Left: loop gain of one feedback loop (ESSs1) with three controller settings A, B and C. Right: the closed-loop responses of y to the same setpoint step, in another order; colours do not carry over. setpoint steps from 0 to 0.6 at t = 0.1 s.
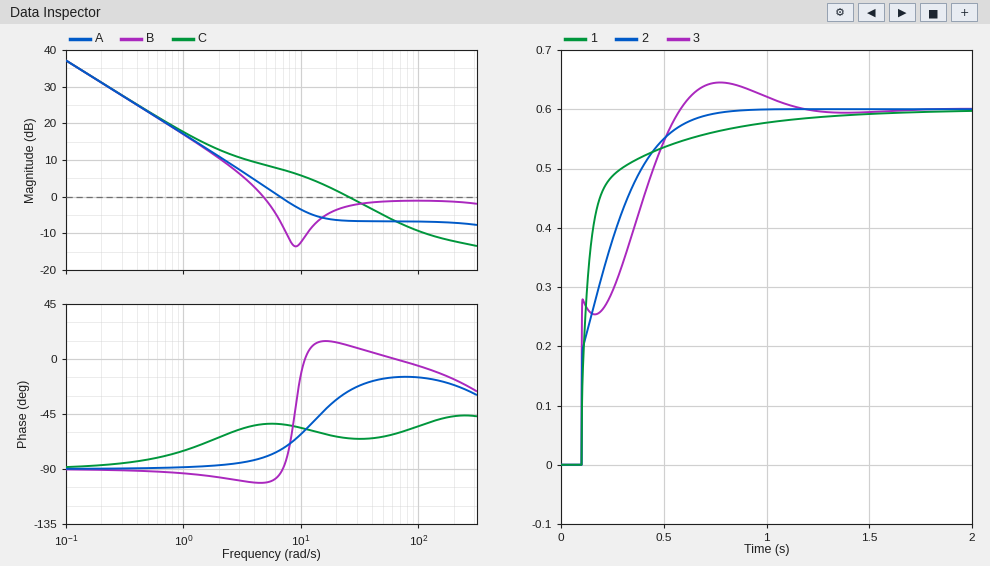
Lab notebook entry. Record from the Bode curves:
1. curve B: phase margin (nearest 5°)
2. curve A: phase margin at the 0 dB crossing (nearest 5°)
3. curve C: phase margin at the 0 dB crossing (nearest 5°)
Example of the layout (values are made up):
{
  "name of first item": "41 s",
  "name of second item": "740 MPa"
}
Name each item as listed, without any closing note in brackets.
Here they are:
{
  "curve B: phase margin": "80°",
  "curve A: phase margin at the 0 dB crossing": "105°",
  "curve C: phase margin at the 0 dB crossing": "115°"
}
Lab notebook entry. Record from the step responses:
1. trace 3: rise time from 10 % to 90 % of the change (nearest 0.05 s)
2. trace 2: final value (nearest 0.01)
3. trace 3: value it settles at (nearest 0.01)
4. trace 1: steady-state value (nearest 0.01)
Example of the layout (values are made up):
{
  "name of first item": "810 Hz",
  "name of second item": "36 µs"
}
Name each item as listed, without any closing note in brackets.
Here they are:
{
  "trace 3: rise time from 10 % to 90 % of the change": "0.40 s",
  "trace 2: final value": "0.60",
  "trace 3: value it settles at": "0.60",
  "trace 1: steady-state value": "0.60"
}
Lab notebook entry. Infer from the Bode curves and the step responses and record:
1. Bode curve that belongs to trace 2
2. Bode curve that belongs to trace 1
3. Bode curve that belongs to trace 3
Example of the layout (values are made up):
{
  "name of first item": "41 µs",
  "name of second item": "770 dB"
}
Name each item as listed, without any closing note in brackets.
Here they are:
{
  "Bode curve that belongs to trace 2": "A",
  "Bode curve that belongs to trace 1": "C",
  "Bode curve that belongs to trace 3": "B"
}
